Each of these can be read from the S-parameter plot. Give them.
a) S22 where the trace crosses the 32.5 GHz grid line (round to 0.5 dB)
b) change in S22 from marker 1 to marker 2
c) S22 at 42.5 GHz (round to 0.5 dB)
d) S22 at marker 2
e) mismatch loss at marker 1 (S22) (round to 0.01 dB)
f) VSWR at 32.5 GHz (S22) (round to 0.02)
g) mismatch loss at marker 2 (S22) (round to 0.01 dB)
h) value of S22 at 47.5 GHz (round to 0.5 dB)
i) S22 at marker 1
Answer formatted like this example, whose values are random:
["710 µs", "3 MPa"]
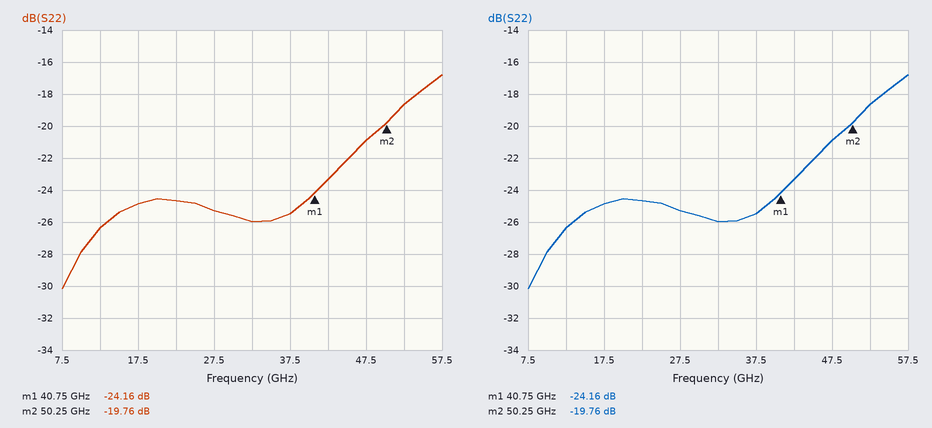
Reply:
["-26.0 dB", "4.40 dB", "-23.5 dB", "-19.76 dB", "0.02 dB", "1.10", "0.05 dB", "-21.0 dB", "-24.16 dB"]
